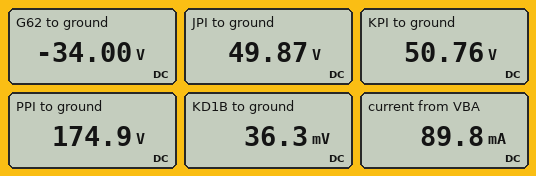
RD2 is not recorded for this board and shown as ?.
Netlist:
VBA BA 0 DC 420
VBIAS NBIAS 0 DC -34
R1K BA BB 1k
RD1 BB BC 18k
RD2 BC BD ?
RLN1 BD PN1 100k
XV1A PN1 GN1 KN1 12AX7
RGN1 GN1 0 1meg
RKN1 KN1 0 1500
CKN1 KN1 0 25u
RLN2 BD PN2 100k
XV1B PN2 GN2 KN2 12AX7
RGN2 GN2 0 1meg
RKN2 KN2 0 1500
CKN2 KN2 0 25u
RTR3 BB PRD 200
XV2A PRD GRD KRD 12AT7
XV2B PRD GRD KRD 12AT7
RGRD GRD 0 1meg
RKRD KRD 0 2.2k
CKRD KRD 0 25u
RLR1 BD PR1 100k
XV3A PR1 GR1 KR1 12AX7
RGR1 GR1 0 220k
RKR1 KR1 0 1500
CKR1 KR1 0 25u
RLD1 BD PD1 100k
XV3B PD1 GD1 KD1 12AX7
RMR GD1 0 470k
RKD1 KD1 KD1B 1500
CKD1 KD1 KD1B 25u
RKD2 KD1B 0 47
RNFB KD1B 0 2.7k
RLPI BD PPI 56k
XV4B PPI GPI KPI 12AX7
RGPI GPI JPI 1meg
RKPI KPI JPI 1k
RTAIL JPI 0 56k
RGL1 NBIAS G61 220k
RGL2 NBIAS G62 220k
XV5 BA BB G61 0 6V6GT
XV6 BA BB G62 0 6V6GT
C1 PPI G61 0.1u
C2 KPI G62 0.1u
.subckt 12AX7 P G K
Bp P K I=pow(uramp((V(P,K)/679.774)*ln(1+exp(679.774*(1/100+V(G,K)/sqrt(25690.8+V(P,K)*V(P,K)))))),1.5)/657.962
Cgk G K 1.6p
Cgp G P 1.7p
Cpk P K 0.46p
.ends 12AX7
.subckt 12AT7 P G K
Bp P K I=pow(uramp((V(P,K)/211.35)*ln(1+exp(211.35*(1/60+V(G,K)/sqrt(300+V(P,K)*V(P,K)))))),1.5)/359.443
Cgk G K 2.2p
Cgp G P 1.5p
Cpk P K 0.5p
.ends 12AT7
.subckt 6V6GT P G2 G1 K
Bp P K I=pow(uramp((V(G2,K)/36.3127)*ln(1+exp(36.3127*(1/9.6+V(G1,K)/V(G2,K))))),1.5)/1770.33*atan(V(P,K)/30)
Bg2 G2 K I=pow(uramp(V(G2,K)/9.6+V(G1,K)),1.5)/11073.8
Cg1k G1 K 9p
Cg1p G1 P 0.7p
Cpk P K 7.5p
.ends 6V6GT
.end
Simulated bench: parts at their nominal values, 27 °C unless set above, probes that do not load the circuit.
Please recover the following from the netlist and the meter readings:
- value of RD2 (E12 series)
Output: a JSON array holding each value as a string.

["27 kΩ"]
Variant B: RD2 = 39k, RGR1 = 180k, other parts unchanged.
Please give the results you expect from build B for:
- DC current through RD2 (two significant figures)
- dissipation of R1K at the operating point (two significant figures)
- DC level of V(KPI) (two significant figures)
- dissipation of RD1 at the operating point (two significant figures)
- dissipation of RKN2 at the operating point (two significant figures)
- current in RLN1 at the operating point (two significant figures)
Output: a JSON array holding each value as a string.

["3.7 mA", "140 mW", "45 V", "240 mW", "770 µW", "720 µA"]
